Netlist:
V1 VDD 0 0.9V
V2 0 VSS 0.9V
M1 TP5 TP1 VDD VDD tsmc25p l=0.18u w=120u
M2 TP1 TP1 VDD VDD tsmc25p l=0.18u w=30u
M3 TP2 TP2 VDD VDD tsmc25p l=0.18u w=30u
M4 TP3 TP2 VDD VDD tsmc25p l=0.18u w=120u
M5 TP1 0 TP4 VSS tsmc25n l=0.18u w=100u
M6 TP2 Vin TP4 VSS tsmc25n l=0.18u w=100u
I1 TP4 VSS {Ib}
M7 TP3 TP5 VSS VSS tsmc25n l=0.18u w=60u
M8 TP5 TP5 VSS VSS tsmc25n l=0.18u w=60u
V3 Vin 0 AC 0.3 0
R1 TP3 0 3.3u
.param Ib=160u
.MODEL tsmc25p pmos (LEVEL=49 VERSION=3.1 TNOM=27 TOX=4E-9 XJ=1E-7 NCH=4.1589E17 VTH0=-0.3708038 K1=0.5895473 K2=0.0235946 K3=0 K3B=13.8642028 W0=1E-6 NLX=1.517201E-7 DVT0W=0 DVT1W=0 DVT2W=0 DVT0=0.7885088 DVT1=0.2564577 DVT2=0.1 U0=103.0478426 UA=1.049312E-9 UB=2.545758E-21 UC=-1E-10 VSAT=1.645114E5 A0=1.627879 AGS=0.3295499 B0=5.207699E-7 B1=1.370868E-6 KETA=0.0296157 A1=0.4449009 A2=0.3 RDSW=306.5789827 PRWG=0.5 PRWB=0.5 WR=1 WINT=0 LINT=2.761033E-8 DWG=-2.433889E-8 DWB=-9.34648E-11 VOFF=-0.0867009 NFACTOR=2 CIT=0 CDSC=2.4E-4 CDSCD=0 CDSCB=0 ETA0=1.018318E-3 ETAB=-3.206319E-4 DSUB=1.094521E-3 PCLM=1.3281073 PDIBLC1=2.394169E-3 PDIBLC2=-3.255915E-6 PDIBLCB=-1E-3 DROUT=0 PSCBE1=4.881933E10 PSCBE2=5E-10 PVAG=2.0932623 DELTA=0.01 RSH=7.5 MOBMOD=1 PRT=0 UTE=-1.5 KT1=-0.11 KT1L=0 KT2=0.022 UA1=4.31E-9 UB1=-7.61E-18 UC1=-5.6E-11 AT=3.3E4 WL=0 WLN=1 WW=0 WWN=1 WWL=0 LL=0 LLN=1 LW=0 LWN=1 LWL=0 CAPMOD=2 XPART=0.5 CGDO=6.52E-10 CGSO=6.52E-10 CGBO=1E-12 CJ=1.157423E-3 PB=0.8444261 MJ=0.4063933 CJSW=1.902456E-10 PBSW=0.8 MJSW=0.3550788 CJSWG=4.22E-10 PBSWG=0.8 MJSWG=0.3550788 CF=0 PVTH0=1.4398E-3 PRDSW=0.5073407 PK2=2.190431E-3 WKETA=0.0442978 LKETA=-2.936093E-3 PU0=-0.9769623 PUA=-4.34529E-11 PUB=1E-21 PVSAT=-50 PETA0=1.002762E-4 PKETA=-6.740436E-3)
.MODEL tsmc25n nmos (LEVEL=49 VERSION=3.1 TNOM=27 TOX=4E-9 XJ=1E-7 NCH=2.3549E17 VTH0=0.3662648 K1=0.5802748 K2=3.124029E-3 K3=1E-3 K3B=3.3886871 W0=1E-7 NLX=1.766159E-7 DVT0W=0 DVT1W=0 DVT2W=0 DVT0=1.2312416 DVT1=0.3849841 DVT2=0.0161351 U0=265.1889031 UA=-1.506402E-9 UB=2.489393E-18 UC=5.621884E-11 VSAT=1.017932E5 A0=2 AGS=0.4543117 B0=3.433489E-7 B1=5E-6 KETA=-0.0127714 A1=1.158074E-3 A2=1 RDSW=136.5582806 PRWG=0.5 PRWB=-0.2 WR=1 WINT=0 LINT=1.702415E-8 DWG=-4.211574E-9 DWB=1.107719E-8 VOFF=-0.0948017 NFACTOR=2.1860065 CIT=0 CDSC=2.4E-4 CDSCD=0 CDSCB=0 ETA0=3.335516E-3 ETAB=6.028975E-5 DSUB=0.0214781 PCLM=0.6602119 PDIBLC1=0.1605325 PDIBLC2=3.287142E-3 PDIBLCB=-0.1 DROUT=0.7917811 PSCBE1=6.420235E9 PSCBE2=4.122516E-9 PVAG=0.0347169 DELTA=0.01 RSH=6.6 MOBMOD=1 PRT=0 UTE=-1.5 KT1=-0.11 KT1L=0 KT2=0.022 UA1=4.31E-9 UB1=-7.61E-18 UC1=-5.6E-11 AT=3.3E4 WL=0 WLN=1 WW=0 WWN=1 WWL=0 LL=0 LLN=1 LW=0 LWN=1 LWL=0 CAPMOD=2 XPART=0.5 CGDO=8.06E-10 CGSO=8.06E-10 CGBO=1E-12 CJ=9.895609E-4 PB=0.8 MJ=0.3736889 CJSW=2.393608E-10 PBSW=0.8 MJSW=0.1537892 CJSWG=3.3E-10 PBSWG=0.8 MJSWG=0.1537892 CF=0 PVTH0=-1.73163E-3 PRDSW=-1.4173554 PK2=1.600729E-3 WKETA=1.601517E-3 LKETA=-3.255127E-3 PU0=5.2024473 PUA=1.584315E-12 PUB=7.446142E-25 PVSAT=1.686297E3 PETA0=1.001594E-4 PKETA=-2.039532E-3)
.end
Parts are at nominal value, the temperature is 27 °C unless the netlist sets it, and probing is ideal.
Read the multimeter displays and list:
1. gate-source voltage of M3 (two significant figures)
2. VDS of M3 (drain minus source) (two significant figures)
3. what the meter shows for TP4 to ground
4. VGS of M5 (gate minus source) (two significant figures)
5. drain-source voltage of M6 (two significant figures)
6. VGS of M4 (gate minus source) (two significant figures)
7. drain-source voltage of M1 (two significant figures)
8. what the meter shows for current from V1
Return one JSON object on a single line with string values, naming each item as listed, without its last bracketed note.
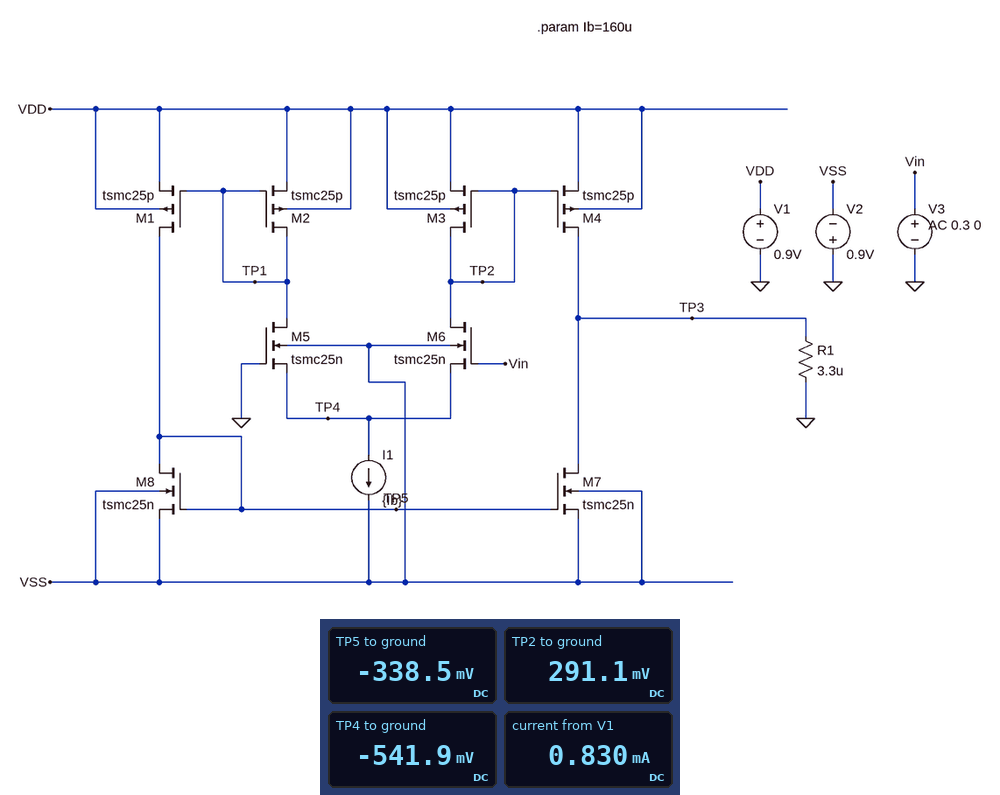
{"gate-source voltage of M3": "-610 mV", "VDS of M3 (drain minus source)": "-610 mV", "what the meter shows for TP4 to ground": "-541.9 mV", "VGS of M5 (gate minus source)": "540 mV", "drain-source voltage of M6": "830 mV", "VGS of M4 (gate minus source)": "-610 mV", "drain-source voltage of M1": "-1.2 V", "what the meter shows for current from V1": "0.830 mA"}
